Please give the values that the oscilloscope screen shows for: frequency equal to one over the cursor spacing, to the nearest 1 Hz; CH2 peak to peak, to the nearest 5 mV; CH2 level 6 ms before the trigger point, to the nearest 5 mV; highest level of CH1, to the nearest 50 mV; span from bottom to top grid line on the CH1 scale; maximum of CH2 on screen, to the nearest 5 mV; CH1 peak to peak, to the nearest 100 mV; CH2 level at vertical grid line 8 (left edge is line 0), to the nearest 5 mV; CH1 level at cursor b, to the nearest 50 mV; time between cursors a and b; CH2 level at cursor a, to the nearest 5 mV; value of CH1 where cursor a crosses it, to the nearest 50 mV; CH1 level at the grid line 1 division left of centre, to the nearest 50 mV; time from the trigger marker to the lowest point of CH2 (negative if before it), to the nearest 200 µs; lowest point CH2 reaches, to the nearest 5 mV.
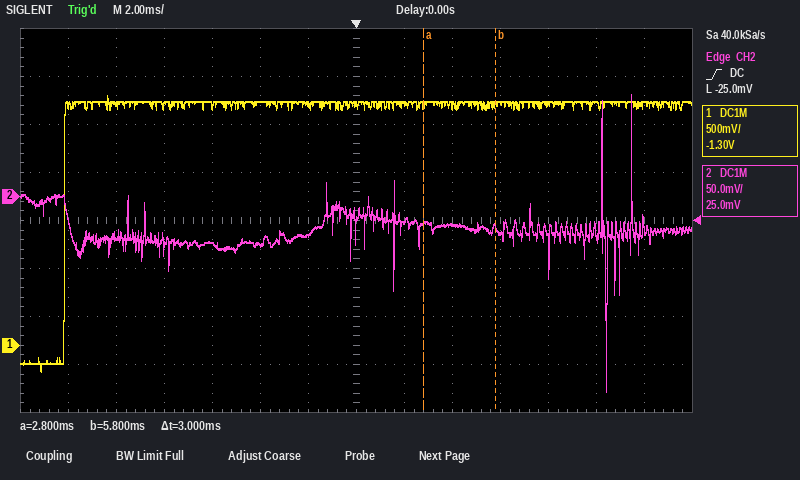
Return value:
333 Hz
310 mV
-50 mV
2.60 V
4 V
105 mV
2.90 V
-25 mV
2.50 V
3 ms
-30 mV
2.50 V
2.50 V
+10.4 ms
-205 mV
